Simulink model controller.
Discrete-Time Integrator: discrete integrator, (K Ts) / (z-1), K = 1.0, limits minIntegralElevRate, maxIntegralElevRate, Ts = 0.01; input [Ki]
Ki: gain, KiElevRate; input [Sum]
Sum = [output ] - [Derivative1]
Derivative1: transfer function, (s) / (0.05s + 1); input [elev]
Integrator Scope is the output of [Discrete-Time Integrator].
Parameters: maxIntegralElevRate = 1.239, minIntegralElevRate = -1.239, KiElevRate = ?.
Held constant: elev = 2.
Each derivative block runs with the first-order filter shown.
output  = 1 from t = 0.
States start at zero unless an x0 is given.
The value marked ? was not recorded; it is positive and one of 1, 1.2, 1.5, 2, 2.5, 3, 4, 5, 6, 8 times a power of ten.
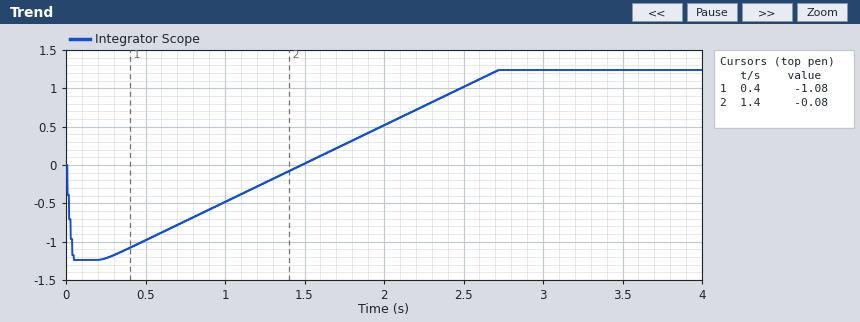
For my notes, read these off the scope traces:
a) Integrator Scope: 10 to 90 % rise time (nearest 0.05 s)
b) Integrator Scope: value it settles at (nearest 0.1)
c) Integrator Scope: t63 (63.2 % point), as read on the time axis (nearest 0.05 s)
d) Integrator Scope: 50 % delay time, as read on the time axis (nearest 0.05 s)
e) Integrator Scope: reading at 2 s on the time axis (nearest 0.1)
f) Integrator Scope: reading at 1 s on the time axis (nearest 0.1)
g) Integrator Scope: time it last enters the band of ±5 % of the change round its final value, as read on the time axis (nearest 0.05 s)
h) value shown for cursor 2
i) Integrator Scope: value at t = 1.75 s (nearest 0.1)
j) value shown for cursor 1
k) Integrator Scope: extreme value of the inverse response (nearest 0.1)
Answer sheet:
1.00 s
1.2
2.25 s
2.10 s
0.5
-0.5
2.65 s
-0.08
0.3
-1.08
-1.2
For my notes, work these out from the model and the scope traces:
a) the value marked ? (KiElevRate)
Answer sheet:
1
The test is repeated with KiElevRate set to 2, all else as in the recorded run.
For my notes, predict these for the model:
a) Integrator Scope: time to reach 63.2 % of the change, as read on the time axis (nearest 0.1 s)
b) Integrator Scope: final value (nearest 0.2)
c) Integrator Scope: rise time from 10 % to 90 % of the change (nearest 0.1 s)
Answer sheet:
1.3 s
1.2
0.5 s
